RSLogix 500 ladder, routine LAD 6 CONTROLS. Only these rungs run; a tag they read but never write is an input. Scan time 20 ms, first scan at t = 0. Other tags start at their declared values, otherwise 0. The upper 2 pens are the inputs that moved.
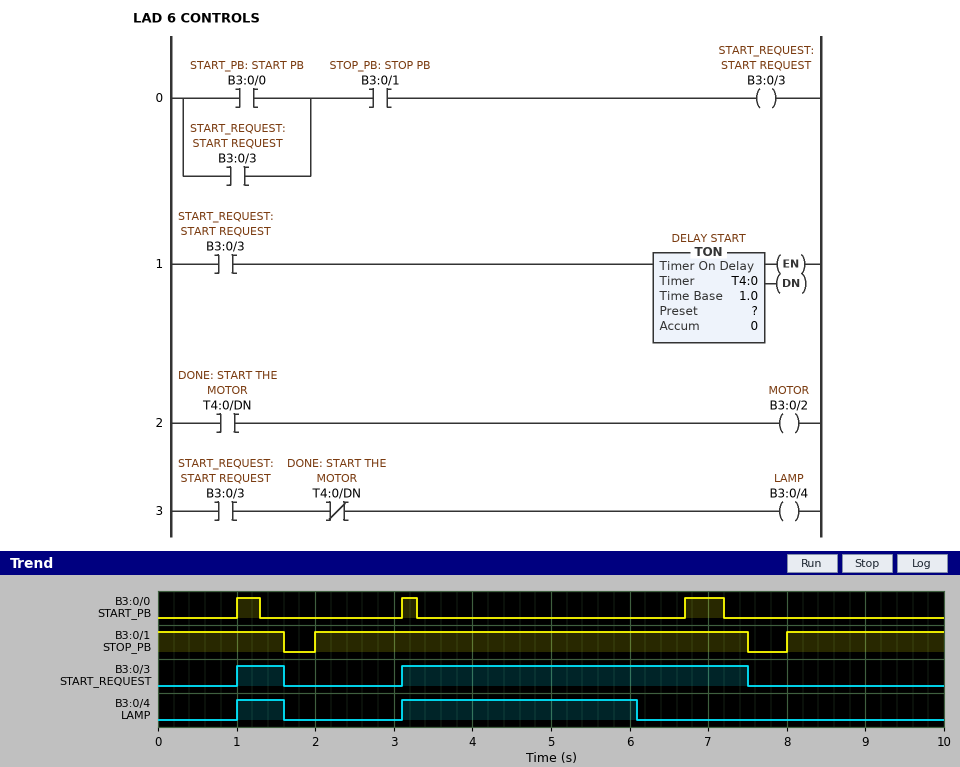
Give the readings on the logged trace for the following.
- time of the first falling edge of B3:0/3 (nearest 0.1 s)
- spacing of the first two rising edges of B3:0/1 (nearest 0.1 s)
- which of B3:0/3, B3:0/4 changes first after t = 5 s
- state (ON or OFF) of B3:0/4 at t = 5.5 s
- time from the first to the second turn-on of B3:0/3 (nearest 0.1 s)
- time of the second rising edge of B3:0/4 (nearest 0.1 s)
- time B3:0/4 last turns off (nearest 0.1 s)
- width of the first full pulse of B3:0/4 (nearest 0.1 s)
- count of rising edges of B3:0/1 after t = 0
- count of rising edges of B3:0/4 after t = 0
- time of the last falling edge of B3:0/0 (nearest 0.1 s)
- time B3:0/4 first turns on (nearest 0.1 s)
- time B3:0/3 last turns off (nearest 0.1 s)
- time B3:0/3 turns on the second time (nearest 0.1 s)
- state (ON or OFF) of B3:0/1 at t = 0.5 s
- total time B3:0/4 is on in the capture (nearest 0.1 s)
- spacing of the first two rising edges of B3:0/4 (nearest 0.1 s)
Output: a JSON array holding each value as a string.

["1.6 s", "6.0 s", "B3:0/4", "ON", "2.1 s", "3.1 s", "6.1 s", "0.6 s", "2", "2", "7.2 s", "1.0 s", "7.5 s", "3.1 s", "ON", "3.6 s", "2.1 s"]
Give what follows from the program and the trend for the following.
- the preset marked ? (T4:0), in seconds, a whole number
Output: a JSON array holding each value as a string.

["3 s"]
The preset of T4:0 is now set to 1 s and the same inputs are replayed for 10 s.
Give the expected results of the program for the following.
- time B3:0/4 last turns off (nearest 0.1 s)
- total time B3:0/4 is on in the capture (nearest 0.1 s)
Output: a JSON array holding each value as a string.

["4.1 s", "1.6 s"]
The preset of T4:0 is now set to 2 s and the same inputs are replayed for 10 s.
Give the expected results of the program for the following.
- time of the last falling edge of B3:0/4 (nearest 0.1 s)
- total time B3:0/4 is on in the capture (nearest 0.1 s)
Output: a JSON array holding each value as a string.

["5.1 s", "2.6 s"]
